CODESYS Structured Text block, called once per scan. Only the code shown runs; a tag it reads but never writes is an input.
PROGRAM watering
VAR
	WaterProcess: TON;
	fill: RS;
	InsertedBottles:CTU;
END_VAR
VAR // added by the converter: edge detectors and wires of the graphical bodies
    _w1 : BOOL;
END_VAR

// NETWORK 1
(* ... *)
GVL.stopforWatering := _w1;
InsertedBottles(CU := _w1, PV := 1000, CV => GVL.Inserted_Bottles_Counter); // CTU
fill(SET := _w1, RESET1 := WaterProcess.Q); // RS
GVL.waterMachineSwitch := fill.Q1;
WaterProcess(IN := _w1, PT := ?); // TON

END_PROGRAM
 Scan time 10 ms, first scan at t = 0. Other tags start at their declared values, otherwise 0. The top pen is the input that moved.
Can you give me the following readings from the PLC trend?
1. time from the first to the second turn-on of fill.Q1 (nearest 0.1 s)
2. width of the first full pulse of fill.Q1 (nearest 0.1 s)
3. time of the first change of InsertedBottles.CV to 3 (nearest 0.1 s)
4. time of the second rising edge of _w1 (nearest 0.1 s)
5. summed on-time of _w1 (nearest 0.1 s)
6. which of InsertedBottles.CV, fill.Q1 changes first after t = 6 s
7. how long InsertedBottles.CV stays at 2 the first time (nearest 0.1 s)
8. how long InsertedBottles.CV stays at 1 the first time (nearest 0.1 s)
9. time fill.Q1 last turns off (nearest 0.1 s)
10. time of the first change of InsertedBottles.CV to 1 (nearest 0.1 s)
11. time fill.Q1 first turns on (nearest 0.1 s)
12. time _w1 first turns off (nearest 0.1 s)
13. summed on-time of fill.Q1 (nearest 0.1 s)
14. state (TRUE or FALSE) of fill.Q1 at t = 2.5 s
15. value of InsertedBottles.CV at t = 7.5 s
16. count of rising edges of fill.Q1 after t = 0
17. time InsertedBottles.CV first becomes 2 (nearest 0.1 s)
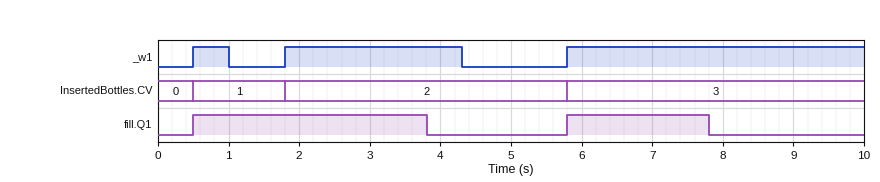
5.3 s
3.3 s
5.8 s
1.8 s
7.2 s
fill.Q1
4.0 s
1.3 s
7.8 s
0.5 s
0.5 s
1.0 s
5.3 s
TRUE
3
2
1.8 s
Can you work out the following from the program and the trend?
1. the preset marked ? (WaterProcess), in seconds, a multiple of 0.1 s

2.0 s
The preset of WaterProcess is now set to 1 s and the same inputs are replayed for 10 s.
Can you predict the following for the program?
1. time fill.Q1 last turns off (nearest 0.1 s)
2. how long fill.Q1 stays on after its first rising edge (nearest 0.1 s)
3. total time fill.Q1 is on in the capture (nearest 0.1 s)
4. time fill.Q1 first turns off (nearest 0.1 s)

6.8 s
2.3 s
3.3 s
2.8 s
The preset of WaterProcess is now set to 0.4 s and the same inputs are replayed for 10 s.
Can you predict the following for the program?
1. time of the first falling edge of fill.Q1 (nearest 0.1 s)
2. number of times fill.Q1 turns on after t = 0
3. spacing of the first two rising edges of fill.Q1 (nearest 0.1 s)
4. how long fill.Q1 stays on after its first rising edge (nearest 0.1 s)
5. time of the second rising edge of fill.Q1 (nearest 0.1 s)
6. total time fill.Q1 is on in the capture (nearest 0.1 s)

0.9 s
3
1.3 s
0.4 s
1.8 s
1.2 s
